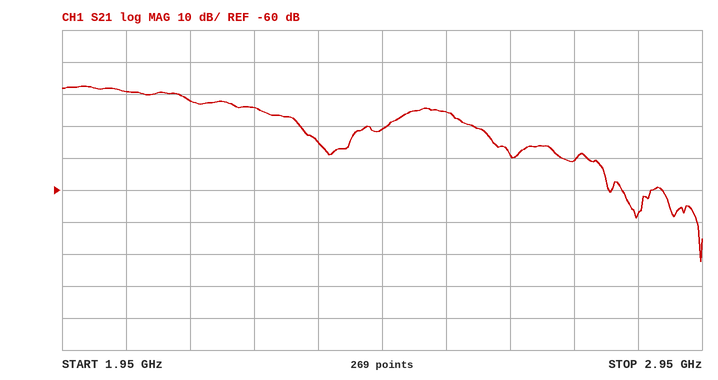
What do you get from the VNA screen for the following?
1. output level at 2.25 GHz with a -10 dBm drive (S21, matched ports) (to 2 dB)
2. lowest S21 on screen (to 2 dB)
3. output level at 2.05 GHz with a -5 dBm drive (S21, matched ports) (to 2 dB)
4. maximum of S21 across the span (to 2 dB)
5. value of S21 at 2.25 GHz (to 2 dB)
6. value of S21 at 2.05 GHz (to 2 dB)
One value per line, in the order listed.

-44 dBm
-82 dB
-34 dBm
-28 dB
-34 dB
-30 dB
